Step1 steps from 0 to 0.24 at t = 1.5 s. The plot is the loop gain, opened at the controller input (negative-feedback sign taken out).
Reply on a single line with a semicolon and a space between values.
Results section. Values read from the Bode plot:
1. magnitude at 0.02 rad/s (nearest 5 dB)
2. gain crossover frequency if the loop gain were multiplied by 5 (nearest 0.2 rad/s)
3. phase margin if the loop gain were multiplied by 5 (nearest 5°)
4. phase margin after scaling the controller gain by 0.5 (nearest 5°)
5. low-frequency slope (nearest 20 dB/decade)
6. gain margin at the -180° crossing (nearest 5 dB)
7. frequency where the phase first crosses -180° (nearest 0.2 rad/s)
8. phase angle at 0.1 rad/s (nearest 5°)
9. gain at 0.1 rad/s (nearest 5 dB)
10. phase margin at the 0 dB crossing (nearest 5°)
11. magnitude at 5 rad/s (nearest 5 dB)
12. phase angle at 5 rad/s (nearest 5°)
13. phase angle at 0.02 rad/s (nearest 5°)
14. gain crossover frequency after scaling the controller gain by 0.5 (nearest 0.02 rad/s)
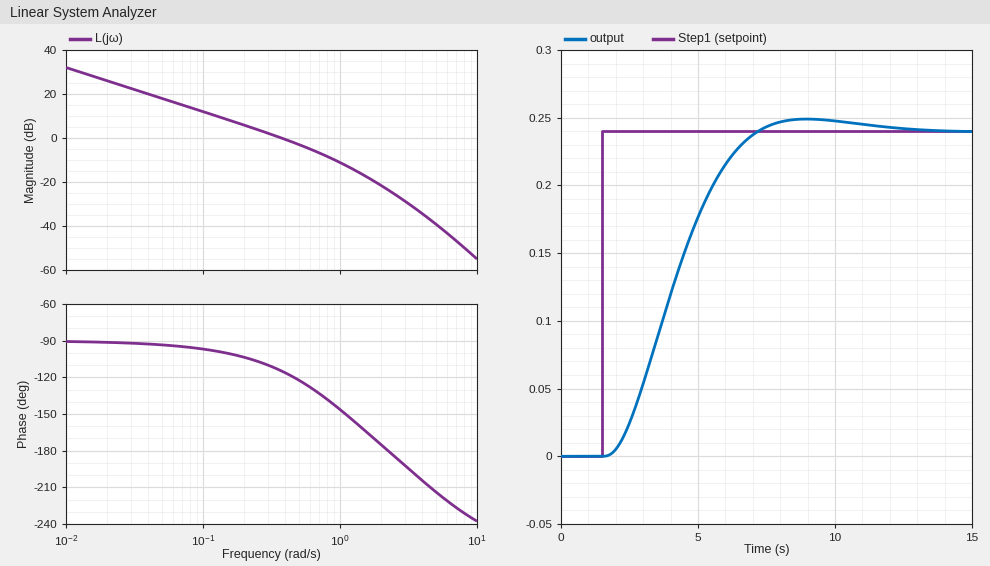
25 dB; 1.2 rad/s; 25°; 75°; -20 dB/decade; 25 dB; 2.2 rad/s; -95°; 10 dB; 65°; -40 dB; -215°; -90°; 0.20 rad/s
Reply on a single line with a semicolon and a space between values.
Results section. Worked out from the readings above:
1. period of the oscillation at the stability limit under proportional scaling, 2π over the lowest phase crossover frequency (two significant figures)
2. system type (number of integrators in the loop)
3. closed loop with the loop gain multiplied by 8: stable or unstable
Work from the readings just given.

2.9 s; 1; stable
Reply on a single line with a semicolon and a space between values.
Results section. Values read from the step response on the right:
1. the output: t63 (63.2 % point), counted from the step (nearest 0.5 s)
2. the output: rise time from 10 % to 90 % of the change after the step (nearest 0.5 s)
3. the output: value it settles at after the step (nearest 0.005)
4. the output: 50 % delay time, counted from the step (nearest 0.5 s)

3.0 s; 3.5 s; 0.240; 2.5 s
